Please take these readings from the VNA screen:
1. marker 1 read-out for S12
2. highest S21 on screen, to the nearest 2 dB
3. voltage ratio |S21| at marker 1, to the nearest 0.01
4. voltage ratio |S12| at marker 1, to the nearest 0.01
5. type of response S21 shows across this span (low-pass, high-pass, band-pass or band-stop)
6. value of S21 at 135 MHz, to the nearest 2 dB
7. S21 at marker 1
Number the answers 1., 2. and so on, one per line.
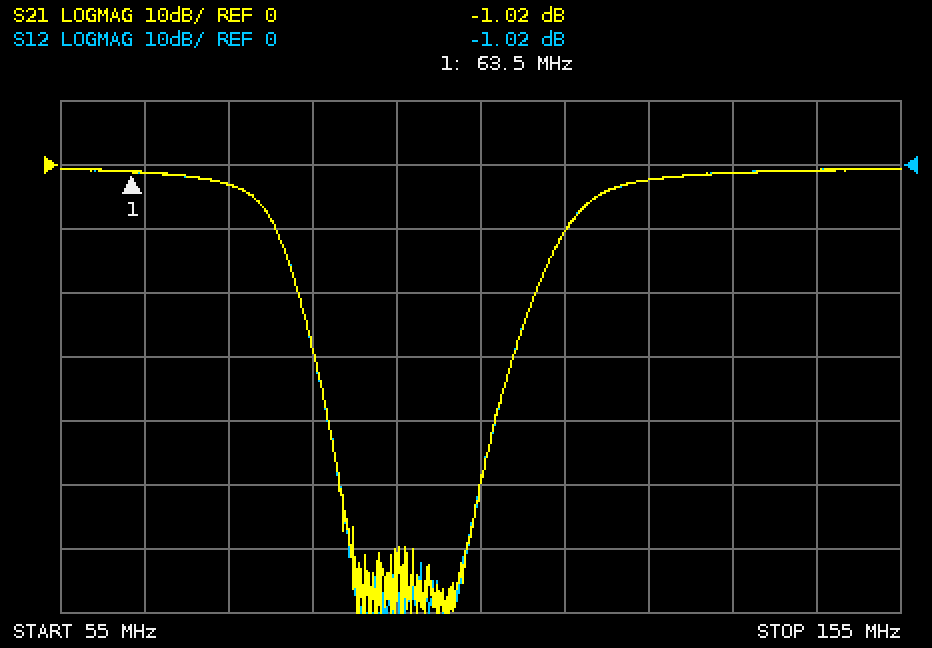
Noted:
1. -1.02 dB
2. 0 dB
3. 0.89
4. 0.89
5. band-stop
6. -2 dB
7. -1.02 dB
